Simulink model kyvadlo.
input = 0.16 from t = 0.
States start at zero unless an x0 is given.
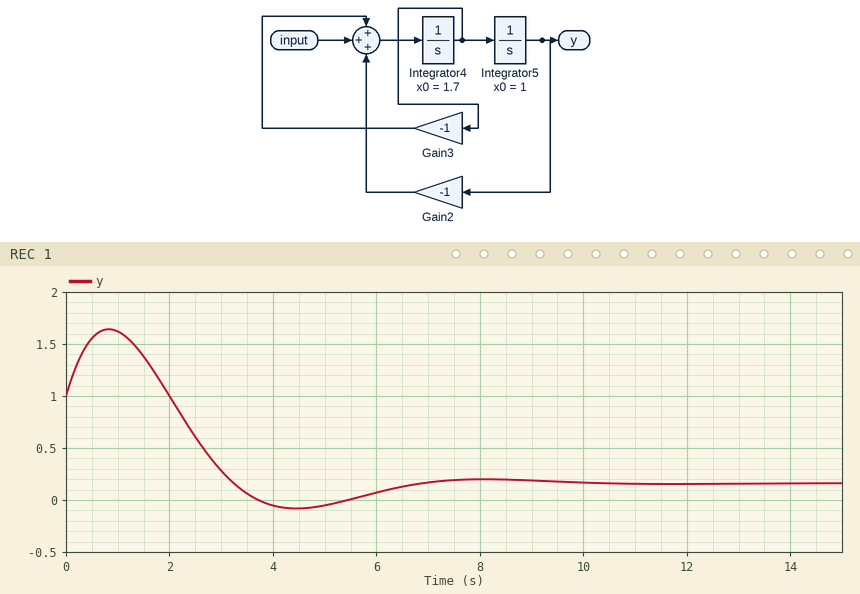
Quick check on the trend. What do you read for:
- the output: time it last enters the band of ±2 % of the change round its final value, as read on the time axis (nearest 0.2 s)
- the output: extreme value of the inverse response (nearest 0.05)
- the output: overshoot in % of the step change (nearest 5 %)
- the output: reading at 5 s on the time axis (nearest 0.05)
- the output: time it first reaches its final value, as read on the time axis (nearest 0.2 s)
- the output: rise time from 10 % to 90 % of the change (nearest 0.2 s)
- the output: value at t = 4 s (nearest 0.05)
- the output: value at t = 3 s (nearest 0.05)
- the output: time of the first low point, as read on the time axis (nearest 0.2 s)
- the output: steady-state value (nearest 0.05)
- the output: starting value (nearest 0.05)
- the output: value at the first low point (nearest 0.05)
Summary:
9.6 s
1.65
30 %
-0.05
3.2 s
1.0 s
-0.05
0.30
4.4 s
0.15
1.00
-0.10
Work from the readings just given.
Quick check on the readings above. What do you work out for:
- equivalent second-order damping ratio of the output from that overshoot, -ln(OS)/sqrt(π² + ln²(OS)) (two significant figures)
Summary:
0.36
